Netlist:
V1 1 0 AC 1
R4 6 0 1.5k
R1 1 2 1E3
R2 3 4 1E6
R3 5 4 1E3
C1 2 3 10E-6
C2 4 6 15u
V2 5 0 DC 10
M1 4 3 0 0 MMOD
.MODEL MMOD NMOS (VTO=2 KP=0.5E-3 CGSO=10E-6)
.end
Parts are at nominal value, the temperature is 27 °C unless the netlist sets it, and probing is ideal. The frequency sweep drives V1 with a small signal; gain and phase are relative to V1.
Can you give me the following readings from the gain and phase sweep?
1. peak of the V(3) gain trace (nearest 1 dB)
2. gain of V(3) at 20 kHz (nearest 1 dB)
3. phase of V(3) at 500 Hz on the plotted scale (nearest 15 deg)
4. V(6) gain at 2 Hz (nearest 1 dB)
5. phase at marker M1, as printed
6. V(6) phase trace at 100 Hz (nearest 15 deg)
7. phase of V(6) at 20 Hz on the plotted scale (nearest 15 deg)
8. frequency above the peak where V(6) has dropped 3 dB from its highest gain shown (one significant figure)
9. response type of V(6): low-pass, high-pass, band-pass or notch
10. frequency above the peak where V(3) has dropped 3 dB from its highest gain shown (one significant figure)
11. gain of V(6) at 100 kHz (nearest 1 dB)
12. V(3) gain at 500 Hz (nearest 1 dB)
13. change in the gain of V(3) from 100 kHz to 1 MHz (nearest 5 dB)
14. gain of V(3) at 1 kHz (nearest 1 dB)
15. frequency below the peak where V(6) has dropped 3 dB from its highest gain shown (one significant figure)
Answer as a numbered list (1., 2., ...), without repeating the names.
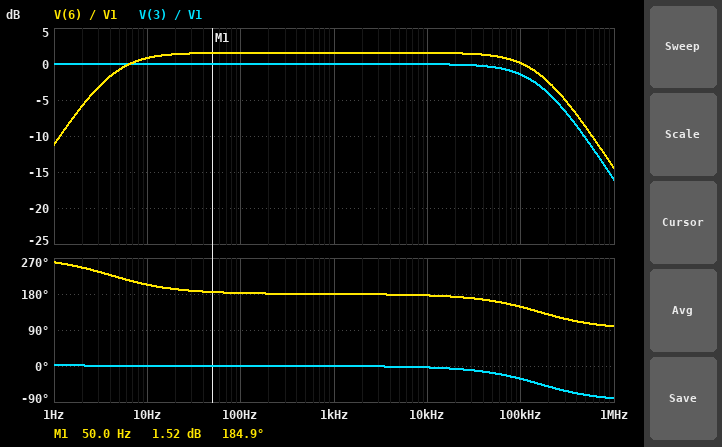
1. 0 dB
2. 0 dB
3. 0 deg
4. -6 dB
5. 184.9 deg
6. 180 deg
7. 195 deg
8. 200 kHz
9. band-pass
10. 200 kHz
11. 0 dB
12. 0 dB
13. -15 dB
14. 0 dB
15. 4 Hz
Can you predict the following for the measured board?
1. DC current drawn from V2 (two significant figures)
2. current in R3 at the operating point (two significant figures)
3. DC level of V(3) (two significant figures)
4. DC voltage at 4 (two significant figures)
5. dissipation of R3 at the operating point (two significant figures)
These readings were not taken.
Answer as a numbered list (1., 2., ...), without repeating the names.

1. 4.0 mA
2. 4.0 mA
3. 6.0 V
4. 6.0 V
5. 16 mW
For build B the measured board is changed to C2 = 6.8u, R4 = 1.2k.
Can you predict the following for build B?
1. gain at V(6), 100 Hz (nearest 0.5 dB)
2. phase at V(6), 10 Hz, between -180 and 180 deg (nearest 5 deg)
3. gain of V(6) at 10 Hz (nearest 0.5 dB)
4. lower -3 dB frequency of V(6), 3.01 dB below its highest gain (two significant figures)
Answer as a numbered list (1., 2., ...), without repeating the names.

1. 0.5 dB
2. -135 deg
3. -2.5 dB
4. 11 Hz
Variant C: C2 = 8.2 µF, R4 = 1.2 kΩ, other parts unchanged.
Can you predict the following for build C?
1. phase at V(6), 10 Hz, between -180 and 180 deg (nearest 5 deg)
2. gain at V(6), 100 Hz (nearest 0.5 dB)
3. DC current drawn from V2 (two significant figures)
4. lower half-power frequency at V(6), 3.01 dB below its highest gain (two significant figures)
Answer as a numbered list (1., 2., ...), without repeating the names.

1. -140 deg
2. 0.5 dB
3. 4.0 mA
4. 8.8 Hz
